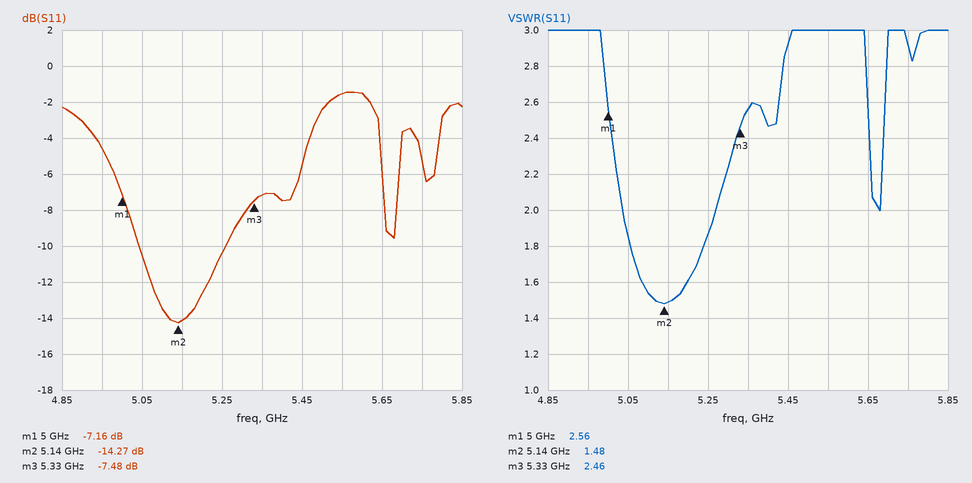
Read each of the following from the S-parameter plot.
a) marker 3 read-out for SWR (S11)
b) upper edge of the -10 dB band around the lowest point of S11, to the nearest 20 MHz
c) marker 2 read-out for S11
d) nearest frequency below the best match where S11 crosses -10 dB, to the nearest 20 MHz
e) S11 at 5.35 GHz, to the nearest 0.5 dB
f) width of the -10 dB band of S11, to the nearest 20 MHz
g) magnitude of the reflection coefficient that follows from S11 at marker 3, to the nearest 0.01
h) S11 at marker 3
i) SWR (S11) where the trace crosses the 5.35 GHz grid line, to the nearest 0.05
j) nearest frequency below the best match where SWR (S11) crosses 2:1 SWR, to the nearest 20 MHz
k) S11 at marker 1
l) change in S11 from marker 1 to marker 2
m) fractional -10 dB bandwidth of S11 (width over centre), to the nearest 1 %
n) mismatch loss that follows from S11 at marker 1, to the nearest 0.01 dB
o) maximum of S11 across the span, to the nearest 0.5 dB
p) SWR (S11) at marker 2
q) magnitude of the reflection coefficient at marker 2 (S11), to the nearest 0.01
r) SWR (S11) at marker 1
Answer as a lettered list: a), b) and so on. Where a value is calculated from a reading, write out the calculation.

a) 2.46
b) 5.26 GHz
c) -14.27 dB
d) 5.04 GHz
e) -7.0 dB
f) 5.26 GHz − 5.04 GHz = 220 MHz
g) 10^(-7.48/20) ≈ 0.42
h) -7.48 dB
i) 2.55
j) 5.04 GHz
k) -7.16 dB
l) -14.27 − (-7.16) = -7.11 dB
m) 220 MHz / 5.15 GHz ≈ 4 %
n) −10 log10(1 − 10^(-7.16/10)) ≈ 0.93 dB
o) -1.5 dB
p) 1.48
q) 10^(-14.27/20) ≈ 0.19
r) 2.56
